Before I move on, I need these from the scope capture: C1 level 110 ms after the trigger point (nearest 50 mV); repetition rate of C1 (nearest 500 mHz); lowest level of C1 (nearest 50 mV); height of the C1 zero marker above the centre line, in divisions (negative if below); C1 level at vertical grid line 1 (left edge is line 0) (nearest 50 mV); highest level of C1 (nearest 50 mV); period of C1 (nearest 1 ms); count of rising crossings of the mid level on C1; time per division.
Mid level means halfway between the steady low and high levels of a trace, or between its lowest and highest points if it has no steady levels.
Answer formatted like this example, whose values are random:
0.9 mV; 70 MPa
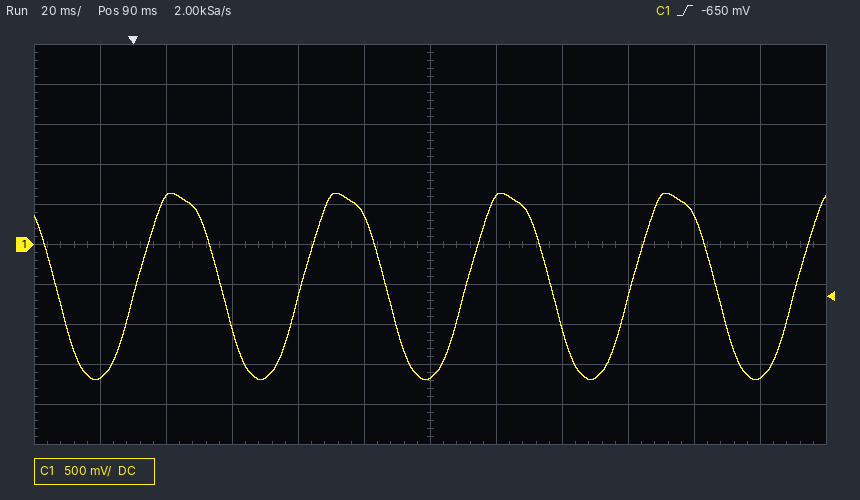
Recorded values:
600 mV; 20.0 Hz; -1.70 V; 0.0 div; -1.65 V; 650 mV; 50 ms; 5; 20 ms
